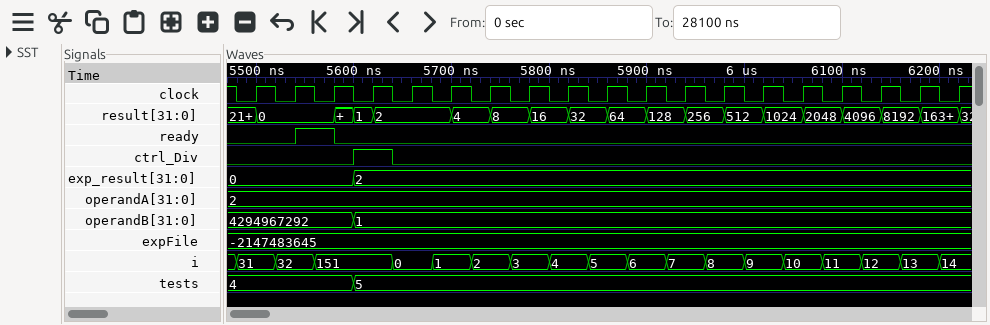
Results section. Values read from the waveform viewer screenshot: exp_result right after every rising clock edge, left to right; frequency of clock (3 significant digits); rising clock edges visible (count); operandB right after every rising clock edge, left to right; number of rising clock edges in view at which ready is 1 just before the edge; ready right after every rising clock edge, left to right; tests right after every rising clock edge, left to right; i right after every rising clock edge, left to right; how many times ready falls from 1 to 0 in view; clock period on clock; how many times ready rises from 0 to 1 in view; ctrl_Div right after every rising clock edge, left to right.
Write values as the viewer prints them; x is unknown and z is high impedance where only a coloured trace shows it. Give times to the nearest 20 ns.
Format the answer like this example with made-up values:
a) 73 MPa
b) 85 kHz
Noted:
a) 0, 0, 0, 2, 2, 2, 2, 2, 2, 2, 2, 2, 2, 2, 2, 2, 2, 2, 2
b) 25.0 MHz
c) 19
d) 4294967292, 4294967292, 4294967292, 1, 1, 1, 1, 1, 1, 1, 1, 1, 1, 1, 1, 1, 1, 1, 1
e) 1
f) 0 1 0 0 0 0 0 0 0 0 0 0 0 0 0 0 0 0 0
g) 4, 4, 4, 5, 5, 5, 5, 5, 5, 5, 5, 5, 5, 5, 5, 5, 5, 5, 5
h) 31, 32, 151, 151, 0, 1, 2, 3, 4, 5, 6, 7, 8, 9, 10, 11, 12, 13, 14
i) 1
j) 40 ns
k) 1
l) 0 0 0 1 0 0 0 0 0 0 0 0 0 0 0 0 0 0 0
